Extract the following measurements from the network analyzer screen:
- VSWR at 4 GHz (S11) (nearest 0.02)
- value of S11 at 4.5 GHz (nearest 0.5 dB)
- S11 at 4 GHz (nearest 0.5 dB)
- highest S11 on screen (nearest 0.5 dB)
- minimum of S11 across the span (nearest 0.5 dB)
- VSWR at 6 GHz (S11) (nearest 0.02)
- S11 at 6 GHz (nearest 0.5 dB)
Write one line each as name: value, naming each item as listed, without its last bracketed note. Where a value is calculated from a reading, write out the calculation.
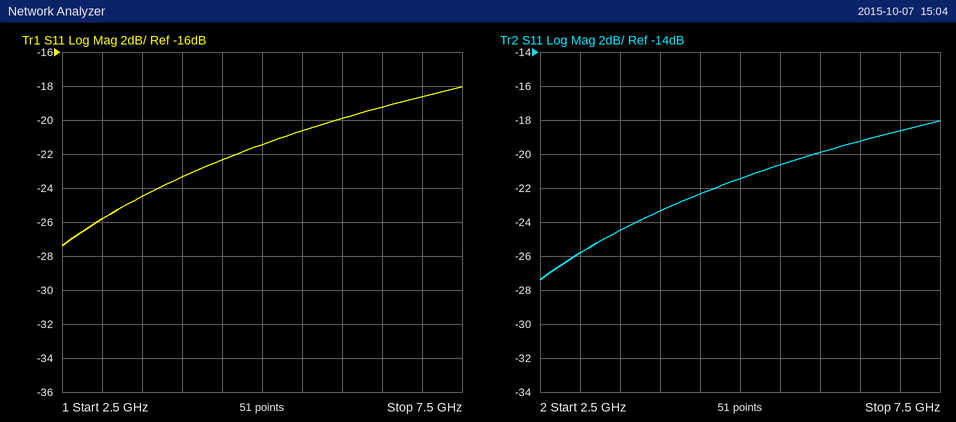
VSWR at 4 GHz (S11): |Γ| = 10^(-23.5/20) = 0.0668; VSWR = (1 + 0.0668)/(1 − 0.0668) ≈ 1.14
value of S11 at 4.5 GHz: -22.5 dB
S11 at 4 GHz: -23.5 dB
highest S11 on screen: -18.0 dB
minimum of S11 across the span: -27.5 dB
VSWR at 6 GHz (S11): |Γ| = 10^(-20/20) = 0.1000; VSWR = (1 + 0.1000)/(1 − 0.1000) ≈ 1.22
S11 at 6 GHz: -20.0 dB
